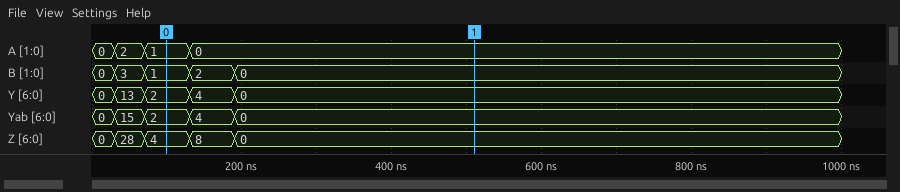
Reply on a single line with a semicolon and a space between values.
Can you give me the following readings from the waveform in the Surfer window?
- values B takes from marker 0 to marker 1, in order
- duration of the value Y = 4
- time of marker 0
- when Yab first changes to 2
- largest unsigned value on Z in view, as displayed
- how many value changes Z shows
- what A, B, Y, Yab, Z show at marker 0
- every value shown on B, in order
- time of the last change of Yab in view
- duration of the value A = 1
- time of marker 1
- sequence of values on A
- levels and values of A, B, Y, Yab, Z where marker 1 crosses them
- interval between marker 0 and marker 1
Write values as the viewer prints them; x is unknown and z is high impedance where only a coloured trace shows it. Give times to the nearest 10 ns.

1, 2, 0; 60 ns; 100 ns; 70 ns; 28; 4; A=1, B=1, Y=2, Yab=2, Z=4; 0, 3, 1, 2, 0; 190 ns; 60 ns; 510 ns; 0, 2, 1, 0; A=0, B=0, Y=0, Yab=0, Z=0; 410 ns
